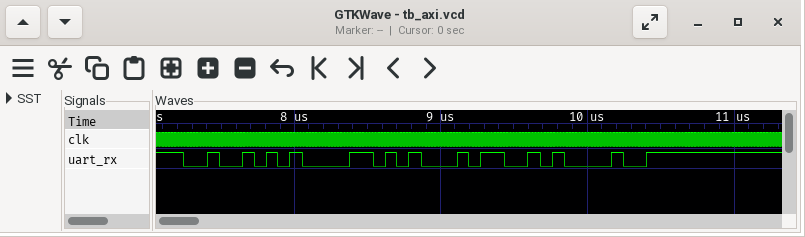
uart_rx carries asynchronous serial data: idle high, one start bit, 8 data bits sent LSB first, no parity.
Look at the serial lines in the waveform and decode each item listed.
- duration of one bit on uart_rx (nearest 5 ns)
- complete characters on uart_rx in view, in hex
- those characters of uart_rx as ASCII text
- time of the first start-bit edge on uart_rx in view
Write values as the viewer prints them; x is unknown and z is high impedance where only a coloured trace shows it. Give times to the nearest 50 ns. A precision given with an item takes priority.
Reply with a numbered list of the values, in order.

1. 80 ns
2. 52, 58, 34, 21
3. "RX4!"
4. 7250 ns
